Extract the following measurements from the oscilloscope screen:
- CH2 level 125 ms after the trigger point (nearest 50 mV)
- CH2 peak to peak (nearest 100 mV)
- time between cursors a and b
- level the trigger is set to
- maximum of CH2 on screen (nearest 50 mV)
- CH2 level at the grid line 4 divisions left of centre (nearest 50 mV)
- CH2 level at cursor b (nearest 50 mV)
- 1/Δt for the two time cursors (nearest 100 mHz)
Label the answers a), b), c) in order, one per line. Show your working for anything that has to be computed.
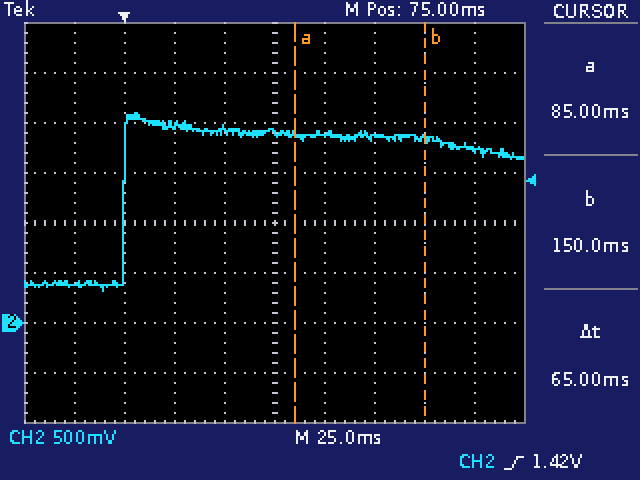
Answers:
a) 1.85 V
b) 1.80 V
c) 65 ms
d) 1.42 V
e) 2.10 V
f) 400 mV
g) 1.85 V
h) 1 / 65 ms ≈ 15.4 Hz
